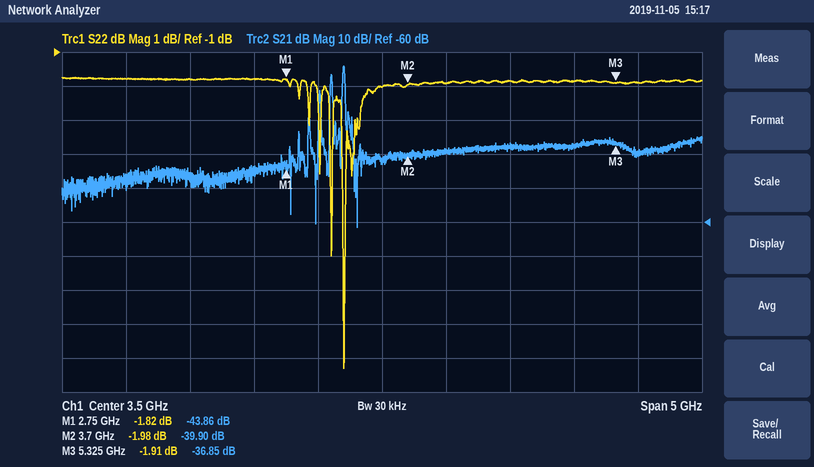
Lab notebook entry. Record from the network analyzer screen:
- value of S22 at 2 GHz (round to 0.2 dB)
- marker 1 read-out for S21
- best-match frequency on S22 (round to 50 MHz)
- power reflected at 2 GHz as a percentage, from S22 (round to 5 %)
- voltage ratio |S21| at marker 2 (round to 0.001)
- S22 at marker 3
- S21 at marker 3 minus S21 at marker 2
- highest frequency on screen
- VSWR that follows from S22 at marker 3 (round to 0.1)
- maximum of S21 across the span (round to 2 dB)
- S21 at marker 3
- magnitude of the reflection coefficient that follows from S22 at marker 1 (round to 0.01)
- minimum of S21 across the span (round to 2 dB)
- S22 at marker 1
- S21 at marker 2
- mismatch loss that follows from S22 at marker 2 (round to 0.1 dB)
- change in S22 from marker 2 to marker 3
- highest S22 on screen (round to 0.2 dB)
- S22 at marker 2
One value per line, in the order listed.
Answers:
-1.8 dB
-43.86 dB
3.20 GHz
65 %
0.010
-1.91 dB
3.05 dB
6 GHz
9.1
-14 dB
-36.85 dB
0.81
-62 dB
-1.82 dB
-39.90 dB
4.4 dB
0.07 dB
-1.8 dB
-1.98 dB
